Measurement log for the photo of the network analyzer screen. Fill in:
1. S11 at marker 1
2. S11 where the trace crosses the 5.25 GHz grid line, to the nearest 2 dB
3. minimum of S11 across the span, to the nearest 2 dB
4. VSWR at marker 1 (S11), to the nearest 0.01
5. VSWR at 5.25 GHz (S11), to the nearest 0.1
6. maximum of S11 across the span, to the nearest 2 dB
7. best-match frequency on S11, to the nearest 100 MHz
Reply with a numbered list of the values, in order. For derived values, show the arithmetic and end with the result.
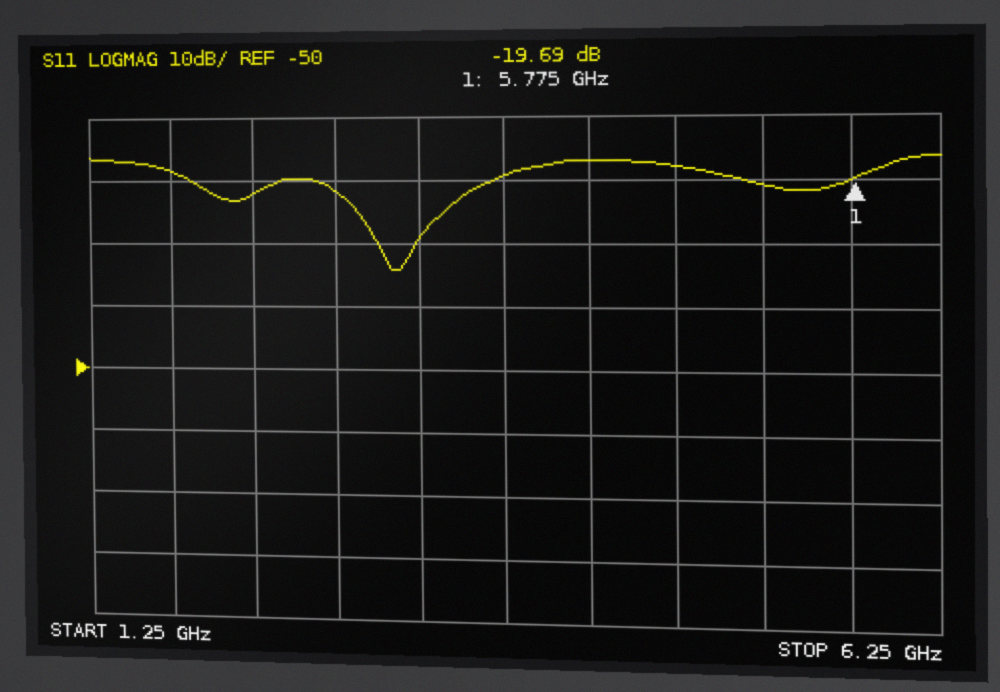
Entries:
1. -19.69 dB
2. -20 dB
3. -34 dB
4. (1 + 0.1036)/(1 − 0.1036) ≈ 1.23
5. |Γ| = 10^(-20/20) = 0.1000; VSWR = (1 + 0.1000)/(1 − 0.1000) ≈ 1.2
6. -16 dB
7. 3.1 GHz
